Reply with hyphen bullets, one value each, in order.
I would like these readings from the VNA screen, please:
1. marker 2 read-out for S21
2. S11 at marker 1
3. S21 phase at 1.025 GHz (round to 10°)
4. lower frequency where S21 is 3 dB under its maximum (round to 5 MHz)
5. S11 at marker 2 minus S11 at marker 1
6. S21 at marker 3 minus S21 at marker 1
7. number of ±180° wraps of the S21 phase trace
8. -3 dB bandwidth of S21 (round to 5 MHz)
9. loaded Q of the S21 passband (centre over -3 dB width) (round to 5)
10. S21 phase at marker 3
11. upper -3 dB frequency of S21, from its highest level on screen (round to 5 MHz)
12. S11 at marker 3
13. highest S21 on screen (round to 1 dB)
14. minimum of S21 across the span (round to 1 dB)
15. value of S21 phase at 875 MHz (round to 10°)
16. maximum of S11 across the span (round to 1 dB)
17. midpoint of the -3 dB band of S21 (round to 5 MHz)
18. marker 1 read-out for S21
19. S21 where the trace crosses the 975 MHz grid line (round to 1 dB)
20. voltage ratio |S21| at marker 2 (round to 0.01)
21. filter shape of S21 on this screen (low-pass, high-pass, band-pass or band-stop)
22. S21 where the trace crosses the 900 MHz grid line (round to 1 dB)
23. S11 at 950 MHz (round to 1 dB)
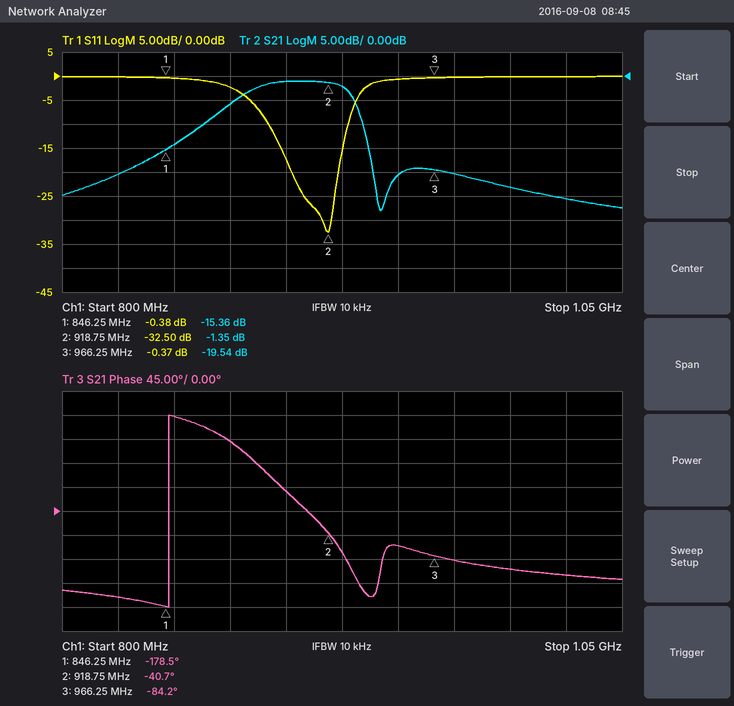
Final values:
- -1.35 dB
- -0.38 dB
- -120°
- 880 MHz
- -32.12 dB
- -4.18 dB
- 1
- 50 MHz
- 20
- -84.2°
- 930 MHz
- -0.37 dB
- -1 dB
- -28 dB
- 130°
- 0 dB
- 905 MHz
- -15.36 dB
- -20 dB
- 0.86
- band-pass
- -1 dB
- -1 dB
